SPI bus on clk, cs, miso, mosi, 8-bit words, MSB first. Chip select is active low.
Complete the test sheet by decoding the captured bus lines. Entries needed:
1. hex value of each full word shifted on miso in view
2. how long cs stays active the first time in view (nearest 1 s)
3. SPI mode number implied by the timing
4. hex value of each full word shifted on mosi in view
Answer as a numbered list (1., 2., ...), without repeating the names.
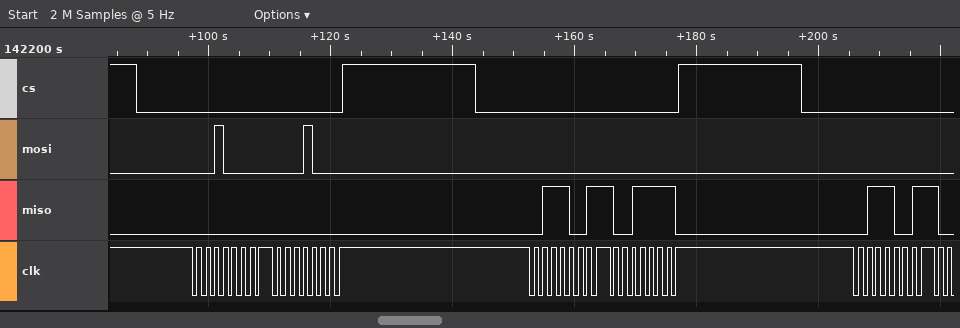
1. 00, 00, 39, 9F, 39
2. 34 s
3. 2
4. 10, 08, 00, 00, 00
